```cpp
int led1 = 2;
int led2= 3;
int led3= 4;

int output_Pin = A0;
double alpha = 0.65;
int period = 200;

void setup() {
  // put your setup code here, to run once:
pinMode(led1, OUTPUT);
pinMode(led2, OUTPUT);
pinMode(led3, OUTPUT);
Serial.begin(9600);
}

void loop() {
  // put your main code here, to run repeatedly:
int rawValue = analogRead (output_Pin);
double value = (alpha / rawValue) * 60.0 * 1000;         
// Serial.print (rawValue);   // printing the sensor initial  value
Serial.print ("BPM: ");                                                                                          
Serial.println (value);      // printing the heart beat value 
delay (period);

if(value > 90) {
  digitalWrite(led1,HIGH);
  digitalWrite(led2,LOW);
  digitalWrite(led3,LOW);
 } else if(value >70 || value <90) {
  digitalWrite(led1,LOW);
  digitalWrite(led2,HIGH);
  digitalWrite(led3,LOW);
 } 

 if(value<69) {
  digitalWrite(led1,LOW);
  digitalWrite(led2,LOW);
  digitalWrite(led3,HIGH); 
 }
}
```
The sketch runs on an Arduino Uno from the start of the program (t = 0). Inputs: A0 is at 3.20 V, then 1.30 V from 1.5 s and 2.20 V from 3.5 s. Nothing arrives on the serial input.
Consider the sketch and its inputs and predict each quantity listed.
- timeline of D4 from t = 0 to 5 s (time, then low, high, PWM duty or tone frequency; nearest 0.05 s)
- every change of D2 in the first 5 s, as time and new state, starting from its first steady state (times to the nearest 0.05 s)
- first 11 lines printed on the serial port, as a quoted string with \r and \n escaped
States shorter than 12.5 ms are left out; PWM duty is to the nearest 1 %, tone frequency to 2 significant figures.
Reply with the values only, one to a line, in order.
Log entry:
0 s low; 0.2 s high; 1.8 s low
0 s low; 1.8 s high; 3.8 s low
"BPM: 59.54\r\nBPM: 59.54\r\nBPM: 59.54\r\nBPM: 59.54\r\nBPM: 59.54\r\nBPM: 59.54\r\nBPM: 59.54\r\nBPM: 59.54\r\nBPM: 146.62\r\nBPM: 146.62\r\nBPM: 146.62\r\n"
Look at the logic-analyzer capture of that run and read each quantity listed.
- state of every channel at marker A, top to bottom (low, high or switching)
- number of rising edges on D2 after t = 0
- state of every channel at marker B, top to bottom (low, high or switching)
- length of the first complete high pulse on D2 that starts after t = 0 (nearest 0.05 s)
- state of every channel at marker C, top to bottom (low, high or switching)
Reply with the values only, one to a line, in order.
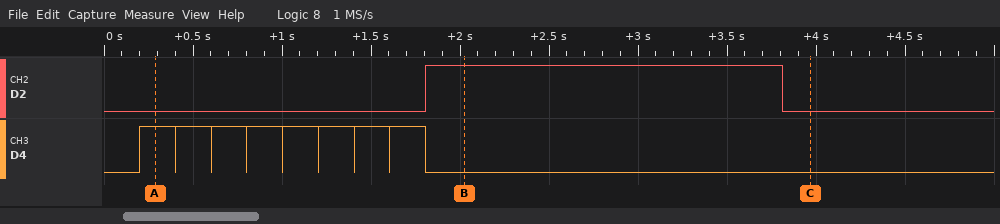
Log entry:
D2 low, D4 high
1
D2 high, D4 low
2.00 s
D2 low, D4 low
